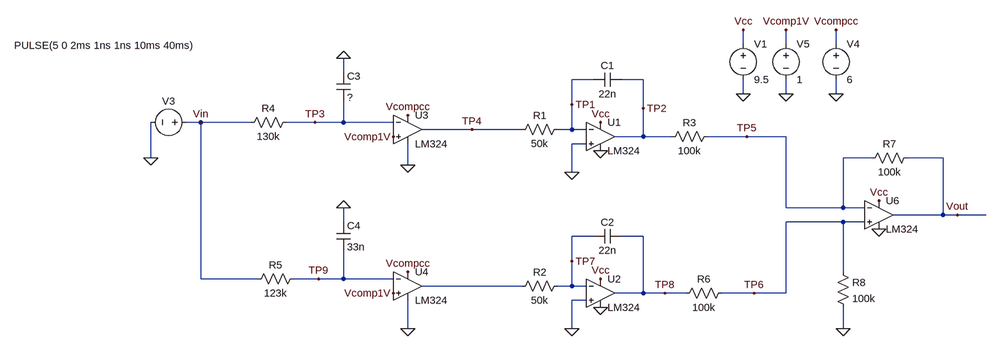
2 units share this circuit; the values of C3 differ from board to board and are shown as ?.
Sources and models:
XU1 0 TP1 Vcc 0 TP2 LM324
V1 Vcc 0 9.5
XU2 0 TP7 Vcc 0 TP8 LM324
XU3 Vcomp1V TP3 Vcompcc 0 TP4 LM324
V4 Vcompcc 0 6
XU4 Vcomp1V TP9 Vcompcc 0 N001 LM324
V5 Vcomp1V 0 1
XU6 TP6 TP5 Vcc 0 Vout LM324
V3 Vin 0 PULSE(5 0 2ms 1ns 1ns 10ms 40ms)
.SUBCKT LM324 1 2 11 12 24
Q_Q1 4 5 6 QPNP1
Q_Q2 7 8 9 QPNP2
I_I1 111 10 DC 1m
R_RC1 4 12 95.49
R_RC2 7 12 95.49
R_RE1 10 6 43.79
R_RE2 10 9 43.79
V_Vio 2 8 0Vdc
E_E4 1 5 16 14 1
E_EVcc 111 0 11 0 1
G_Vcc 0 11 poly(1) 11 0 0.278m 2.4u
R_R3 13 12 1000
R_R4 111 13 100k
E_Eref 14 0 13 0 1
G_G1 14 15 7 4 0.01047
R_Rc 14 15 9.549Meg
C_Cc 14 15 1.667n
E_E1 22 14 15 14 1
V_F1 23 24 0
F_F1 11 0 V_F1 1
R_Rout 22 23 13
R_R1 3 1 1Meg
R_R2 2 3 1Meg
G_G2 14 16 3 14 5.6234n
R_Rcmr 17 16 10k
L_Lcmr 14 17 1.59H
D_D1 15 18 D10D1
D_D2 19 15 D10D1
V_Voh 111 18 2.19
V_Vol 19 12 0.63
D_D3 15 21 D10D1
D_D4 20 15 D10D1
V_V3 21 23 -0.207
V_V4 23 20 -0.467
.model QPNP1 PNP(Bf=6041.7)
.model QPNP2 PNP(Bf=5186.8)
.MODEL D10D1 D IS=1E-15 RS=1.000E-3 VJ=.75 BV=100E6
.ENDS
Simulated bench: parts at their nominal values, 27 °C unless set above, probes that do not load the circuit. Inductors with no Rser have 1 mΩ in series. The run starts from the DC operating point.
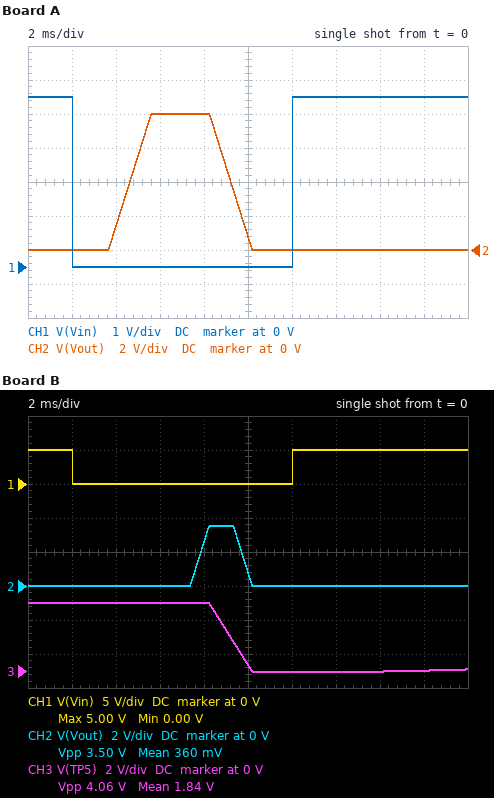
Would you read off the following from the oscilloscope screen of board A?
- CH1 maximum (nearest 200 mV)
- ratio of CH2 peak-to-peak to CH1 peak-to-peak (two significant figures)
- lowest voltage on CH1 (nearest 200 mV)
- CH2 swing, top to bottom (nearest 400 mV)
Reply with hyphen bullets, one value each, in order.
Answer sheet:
- 5.0 V
- 1.6
- 0 V
- 8.0 V
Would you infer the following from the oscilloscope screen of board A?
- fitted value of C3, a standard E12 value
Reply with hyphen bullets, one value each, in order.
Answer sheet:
- 8.2 nF
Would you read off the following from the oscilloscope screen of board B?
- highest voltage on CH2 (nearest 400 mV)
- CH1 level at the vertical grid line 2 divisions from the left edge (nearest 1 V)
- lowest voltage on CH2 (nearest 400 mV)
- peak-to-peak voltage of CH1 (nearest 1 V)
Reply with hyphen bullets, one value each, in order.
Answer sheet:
- 3.6 V
- 0 V
- 0 V
- 5 V
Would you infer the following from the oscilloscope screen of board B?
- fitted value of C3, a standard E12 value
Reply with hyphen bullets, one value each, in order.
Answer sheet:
- 27 nF
